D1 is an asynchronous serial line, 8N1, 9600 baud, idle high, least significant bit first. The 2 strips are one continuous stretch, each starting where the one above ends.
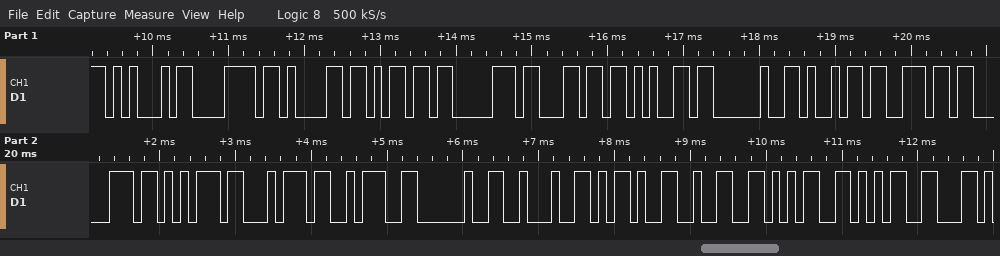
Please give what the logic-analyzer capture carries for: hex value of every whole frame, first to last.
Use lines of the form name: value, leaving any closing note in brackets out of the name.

hex value of every whole frame, first to last: 0x45 0x78 0x61 0x6D 0x70 0x6C 0x65 0x20 0x69 0x6E 0x70 0x75 0x74 0x3A 0x20 0x22 0x2D 0x32 0x35 0x35
